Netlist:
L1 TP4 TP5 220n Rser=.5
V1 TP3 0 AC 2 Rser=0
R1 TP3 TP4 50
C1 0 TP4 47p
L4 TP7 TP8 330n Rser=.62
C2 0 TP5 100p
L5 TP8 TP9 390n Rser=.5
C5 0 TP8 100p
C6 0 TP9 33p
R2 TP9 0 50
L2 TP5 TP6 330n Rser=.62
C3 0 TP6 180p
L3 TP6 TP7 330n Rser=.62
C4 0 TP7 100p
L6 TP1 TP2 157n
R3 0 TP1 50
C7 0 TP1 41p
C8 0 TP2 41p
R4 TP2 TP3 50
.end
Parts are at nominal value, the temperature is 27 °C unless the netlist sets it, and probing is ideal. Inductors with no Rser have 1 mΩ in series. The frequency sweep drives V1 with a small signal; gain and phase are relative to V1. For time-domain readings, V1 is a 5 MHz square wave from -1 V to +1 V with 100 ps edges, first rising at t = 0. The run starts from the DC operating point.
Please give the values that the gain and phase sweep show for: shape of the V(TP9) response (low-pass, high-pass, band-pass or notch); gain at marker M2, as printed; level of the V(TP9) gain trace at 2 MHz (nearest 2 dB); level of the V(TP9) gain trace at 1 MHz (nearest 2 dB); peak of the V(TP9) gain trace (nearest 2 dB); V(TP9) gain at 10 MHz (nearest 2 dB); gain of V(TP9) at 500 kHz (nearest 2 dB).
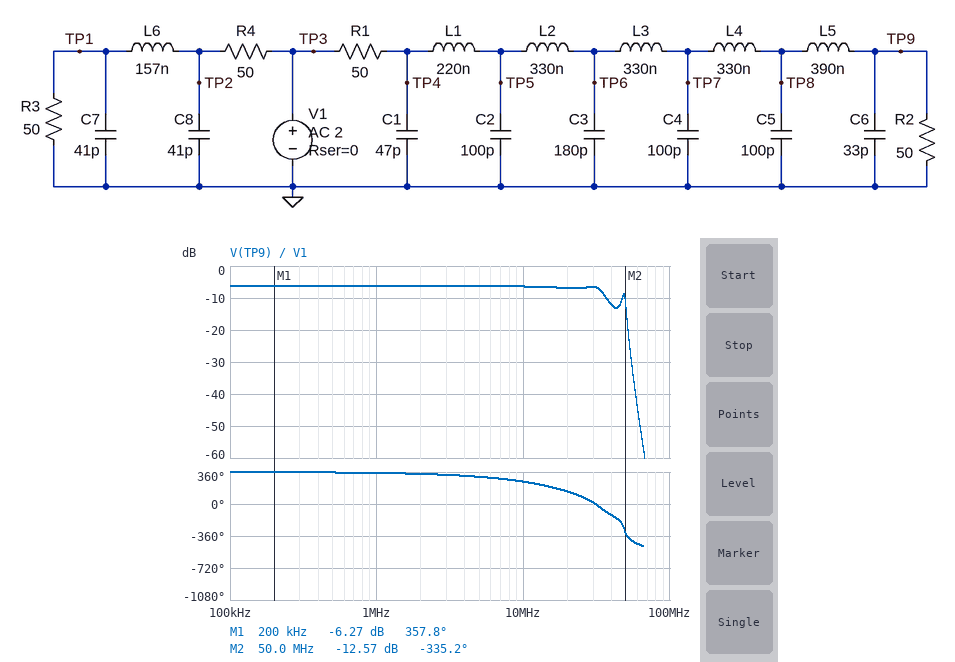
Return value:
low-pass
-12.57 dB
-6 dB
-6 dB
-6 dB
-6 dB
-6 dB
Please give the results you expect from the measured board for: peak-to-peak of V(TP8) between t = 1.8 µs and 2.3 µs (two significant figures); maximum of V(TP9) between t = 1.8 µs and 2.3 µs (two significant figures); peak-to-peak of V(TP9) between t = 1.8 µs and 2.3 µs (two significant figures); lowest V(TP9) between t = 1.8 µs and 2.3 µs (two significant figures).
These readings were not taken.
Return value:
1.6 V
620 mV
1.2 V
-620 mV
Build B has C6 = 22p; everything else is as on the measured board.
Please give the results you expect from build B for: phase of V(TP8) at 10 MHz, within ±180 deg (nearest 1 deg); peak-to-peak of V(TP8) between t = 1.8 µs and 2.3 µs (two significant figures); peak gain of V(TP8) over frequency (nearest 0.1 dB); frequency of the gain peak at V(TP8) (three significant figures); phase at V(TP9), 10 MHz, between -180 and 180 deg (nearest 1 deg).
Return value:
-81 deg
1.7 V
-0.9 dB
48.4 MHz
-108 deg
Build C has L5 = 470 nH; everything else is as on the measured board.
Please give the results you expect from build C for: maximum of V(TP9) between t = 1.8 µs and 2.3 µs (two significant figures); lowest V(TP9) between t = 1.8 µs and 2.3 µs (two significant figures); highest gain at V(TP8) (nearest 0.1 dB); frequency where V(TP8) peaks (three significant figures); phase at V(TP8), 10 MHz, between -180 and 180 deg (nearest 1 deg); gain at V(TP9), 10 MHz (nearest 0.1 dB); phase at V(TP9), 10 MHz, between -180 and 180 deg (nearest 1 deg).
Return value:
600 mV
-600 mV
1.3 dB
48.3 MHz
-80 deg
-6.5 dB
-112 deg
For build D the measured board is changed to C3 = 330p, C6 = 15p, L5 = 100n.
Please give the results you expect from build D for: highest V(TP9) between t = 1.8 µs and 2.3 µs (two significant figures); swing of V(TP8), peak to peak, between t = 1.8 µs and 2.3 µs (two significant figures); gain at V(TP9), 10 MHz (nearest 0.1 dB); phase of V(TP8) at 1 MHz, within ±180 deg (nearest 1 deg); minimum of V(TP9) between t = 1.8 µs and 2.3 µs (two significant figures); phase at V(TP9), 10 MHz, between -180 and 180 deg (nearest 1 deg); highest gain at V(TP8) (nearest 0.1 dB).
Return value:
520 mV
1.1 V
-6.6 dB
-10 deg
-520 mV
-111 deg
-6.2 dB
